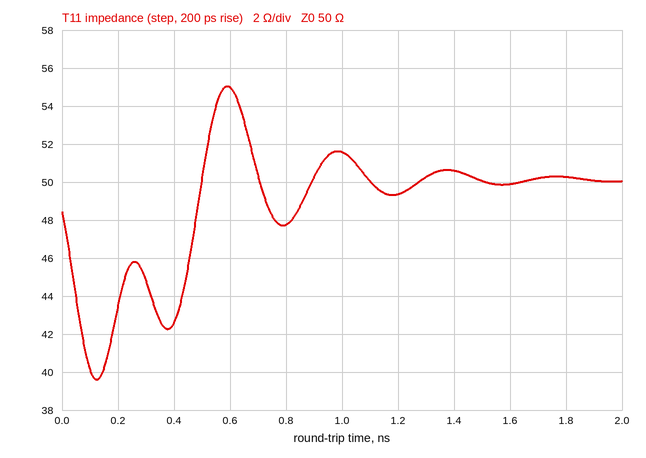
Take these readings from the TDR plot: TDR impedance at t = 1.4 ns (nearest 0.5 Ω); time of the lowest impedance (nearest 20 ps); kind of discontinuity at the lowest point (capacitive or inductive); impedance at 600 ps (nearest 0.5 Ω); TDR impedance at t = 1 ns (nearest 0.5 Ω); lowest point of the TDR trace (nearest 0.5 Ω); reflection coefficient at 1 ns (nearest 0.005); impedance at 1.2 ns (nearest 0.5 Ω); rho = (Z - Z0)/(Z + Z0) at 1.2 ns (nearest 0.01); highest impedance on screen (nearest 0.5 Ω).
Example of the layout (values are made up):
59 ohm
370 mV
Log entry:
50.5 Ω
120 ps
capacitive
55.0 Ω
51.5 Ω
39.5 Ω
+0.015
49.5 Ω
-0.01
55.0 Ω
